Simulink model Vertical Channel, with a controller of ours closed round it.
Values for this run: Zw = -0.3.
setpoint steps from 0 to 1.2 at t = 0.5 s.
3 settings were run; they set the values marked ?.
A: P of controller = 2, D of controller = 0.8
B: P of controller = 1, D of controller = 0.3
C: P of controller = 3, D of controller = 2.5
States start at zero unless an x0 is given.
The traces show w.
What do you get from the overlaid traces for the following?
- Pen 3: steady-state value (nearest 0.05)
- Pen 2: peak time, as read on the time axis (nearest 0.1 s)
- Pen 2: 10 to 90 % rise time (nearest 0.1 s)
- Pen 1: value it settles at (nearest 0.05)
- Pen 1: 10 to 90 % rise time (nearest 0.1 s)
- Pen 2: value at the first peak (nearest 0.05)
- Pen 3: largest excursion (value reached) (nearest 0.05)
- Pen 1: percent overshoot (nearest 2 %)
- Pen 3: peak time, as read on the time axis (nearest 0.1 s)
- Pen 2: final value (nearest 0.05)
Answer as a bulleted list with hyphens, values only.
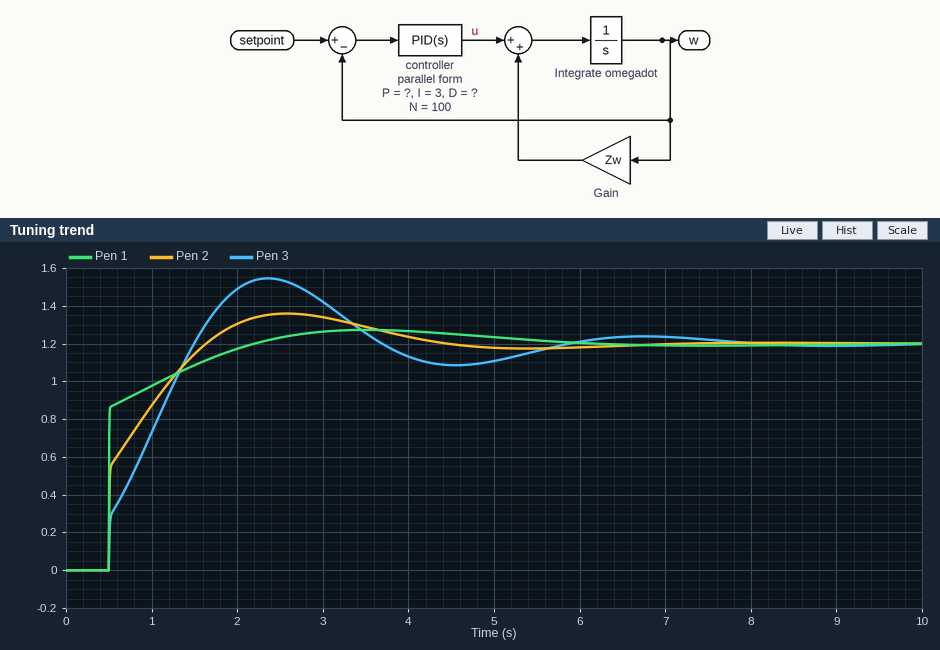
- 1.20
- 2.6 s
- 0.9 s
- 1.20
- 1.0 s
- 1.35
- 1.55
- 6 %
- 2.4 s
- 1.20
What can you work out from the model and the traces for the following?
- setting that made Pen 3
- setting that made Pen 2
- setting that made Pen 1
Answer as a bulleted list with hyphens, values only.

- B
- A
- C
